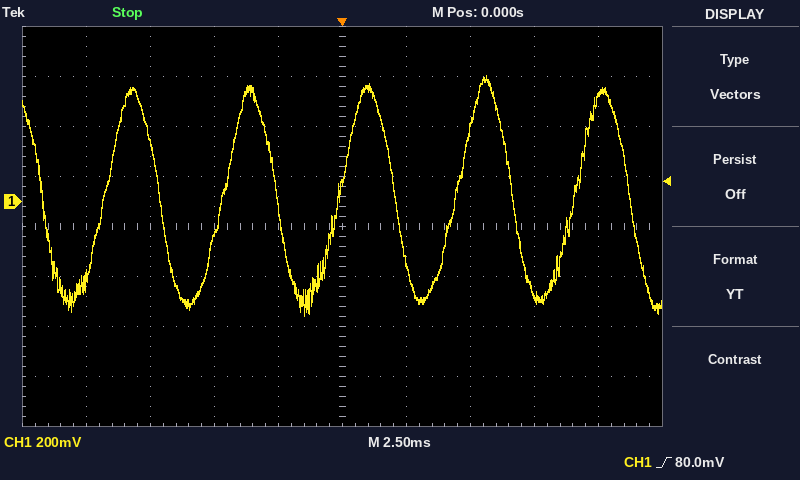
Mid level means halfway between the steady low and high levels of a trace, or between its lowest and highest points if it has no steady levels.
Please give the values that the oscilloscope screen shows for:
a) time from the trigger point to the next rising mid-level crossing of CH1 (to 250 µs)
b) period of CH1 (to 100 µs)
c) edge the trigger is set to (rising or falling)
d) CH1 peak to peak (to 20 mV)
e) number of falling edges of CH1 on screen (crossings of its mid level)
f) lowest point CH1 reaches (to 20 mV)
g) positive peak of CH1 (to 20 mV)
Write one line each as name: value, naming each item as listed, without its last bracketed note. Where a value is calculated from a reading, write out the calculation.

time from the trigger point to the next rising mid-level crossing of CH1: 4.50 ms
period of CH1: 4.6 ms
edge the trigger is set to: rising
CH1 peak to peak: 500 mV − (-460 mV) = 960 mV
number of falling edges of CH1 on screen: 6
lowest point CH1 reaches: -460 mV
positive peak of CH1: 500 mV
